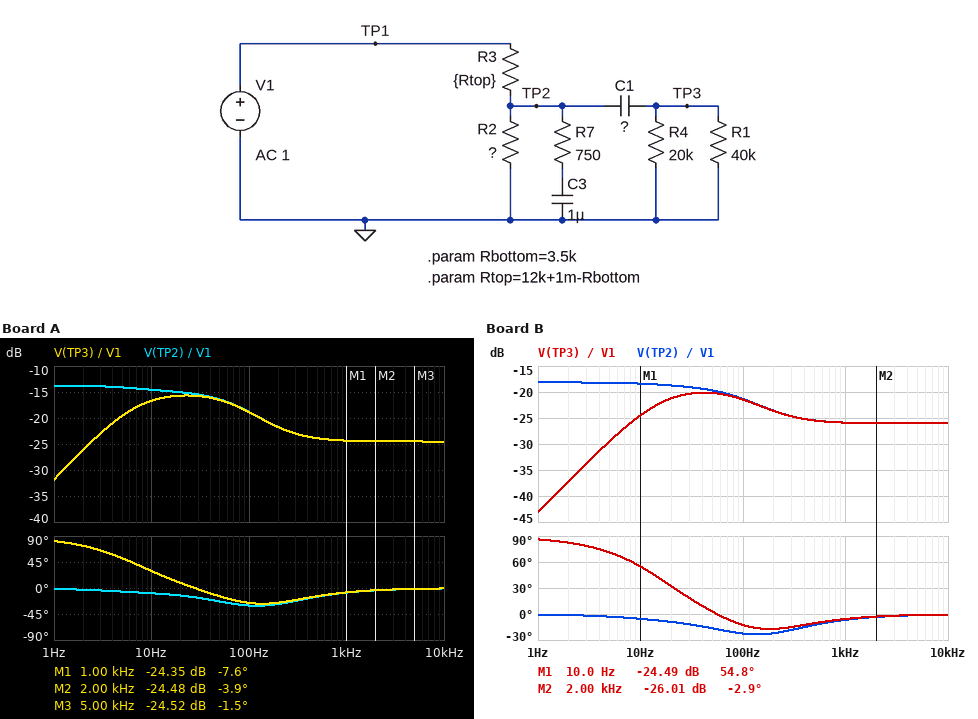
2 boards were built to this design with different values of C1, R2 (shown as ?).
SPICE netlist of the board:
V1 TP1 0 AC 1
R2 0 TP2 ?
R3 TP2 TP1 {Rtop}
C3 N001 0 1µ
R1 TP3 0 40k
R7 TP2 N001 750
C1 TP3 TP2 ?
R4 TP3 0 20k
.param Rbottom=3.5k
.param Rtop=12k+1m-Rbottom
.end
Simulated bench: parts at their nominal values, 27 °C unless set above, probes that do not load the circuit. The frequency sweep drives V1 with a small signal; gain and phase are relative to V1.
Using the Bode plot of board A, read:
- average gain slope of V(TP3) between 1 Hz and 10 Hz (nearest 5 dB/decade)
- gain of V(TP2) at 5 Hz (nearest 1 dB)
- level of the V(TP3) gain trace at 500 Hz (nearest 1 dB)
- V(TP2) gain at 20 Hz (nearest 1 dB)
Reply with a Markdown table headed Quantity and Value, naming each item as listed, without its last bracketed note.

| Quantity | Value |
|---|---|
| average gain slope of V(TP3) between 1 Hz and 10 Hz | 15 dB/decade |
| gain of V(TP2) at 5 Hz | -14 dB |
| level of the V(TP3) gain trace at 500 Hz | -24 dB |
| V(TP2) gain at 20 Hz | -15 dB |
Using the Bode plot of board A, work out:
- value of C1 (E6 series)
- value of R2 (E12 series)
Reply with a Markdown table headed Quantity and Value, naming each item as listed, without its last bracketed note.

| Quantity | Value |
|---|---|
| value of C1 | 1.5 µF |
| value of R2 | 2.2 kΩ |
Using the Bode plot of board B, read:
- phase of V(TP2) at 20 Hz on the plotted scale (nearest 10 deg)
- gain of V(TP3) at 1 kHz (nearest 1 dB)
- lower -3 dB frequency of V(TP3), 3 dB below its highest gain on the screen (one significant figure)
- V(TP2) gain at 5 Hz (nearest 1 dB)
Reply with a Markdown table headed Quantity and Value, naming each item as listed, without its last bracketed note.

| Quantity | Value |
|---|---|
| phase of V(TP2) at 20 Hz on the plotted scale | -10 deg |
| gain of V(TP3) at 1 kHz | -26 dB |
| lower -3 dB frequency of V(TP3), 3 dB below its highest gain on the screen | 10 Hz |
| V(TP2) gain at 5 Hz | -18 dB |
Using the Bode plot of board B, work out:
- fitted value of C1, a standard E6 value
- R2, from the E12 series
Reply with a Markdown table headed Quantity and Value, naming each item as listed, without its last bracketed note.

| Quantity | Value |
|---|---|
| fitted value of C1, a standard E6 value | 680 nF |
| R2, from the E12 series | 1.2 kΩ |
